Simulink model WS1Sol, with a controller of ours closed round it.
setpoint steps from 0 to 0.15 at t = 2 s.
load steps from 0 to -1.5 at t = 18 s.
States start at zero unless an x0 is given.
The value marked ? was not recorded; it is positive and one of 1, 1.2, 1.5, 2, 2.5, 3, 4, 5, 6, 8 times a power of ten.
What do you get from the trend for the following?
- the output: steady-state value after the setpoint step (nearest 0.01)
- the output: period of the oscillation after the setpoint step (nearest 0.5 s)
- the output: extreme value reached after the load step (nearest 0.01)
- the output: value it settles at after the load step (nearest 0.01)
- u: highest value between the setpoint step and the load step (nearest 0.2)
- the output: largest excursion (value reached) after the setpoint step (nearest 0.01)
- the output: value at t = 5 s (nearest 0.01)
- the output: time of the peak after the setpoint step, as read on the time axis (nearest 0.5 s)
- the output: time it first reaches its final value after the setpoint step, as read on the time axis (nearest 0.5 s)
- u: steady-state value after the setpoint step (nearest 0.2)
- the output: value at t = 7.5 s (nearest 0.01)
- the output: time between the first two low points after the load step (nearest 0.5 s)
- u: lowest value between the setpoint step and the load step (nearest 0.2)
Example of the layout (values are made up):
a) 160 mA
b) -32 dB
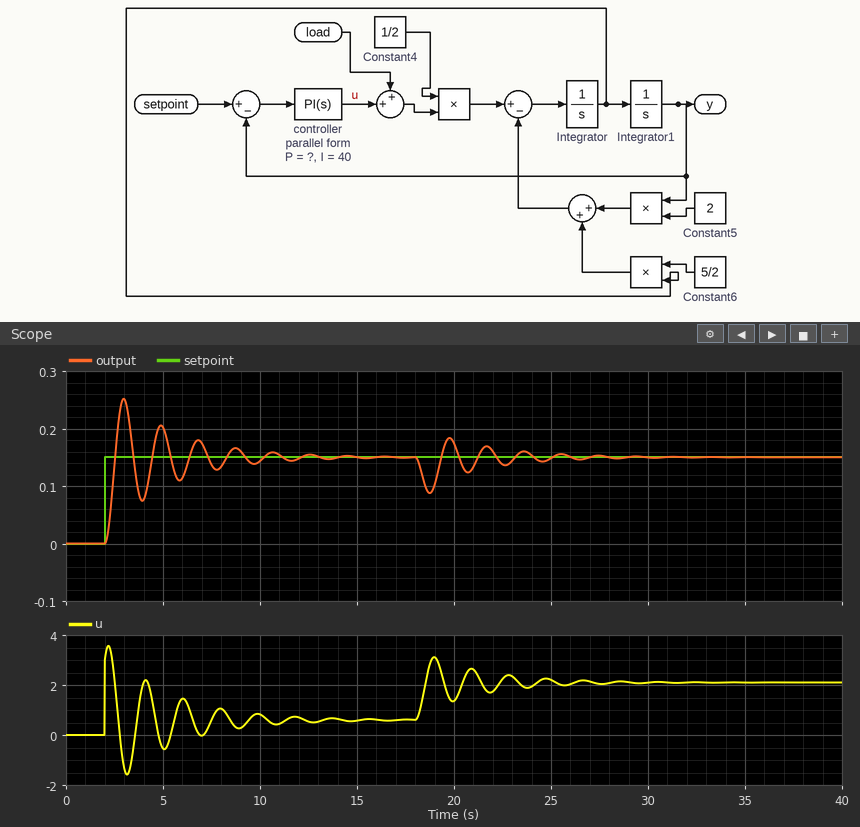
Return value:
a) 0.15
b) 2.0 s
c) 0.09
d) 0.15
e) 3.6
f) 0.25
g) 0.20
h) 3.0 s
i) 2.5 s
j) 0.6
k) 0.14
l) 2.0 s
m) -1.6
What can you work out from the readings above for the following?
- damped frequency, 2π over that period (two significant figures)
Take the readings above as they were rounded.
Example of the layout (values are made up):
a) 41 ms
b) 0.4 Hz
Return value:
a) 3.1 rad/s
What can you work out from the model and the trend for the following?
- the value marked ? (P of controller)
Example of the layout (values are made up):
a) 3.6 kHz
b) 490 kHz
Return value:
a) 20
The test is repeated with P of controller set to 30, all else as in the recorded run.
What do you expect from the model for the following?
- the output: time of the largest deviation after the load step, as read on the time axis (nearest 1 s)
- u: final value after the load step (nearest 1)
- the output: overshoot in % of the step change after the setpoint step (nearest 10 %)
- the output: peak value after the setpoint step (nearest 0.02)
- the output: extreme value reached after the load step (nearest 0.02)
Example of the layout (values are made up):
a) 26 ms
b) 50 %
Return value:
a) 19 s
b) 2
c) 60 %
d) 0.24
e) 0.10
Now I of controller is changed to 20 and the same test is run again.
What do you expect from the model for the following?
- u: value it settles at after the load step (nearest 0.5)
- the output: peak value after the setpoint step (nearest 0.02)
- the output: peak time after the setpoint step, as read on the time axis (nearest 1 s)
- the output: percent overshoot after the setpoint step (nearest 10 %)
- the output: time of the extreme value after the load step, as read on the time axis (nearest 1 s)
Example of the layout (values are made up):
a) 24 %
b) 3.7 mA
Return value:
a) 2.0
b) 0.22
c) 3 s
d) 40 %
e) 19 s
